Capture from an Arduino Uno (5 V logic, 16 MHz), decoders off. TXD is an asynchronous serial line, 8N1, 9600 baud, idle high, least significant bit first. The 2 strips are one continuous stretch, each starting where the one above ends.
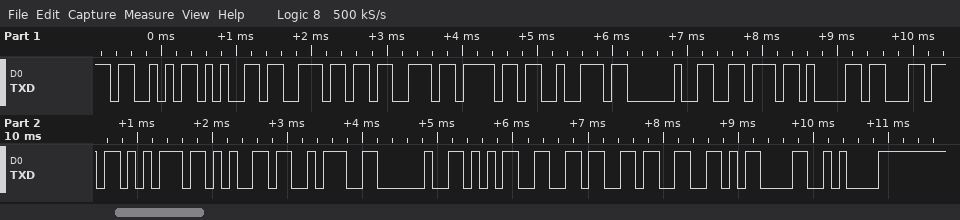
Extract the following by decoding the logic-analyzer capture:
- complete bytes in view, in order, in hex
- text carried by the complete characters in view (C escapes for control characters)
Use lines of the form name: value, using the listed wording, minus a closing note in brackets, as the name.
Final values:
complete bytes in view, in order, in hex: 53 65 6E 73 6F 72 20 76 61 6C 75 65 3A 20 35 36 33 0D 0A
text carried by the complete characters in view: "Sensor value: 563\r\n"
